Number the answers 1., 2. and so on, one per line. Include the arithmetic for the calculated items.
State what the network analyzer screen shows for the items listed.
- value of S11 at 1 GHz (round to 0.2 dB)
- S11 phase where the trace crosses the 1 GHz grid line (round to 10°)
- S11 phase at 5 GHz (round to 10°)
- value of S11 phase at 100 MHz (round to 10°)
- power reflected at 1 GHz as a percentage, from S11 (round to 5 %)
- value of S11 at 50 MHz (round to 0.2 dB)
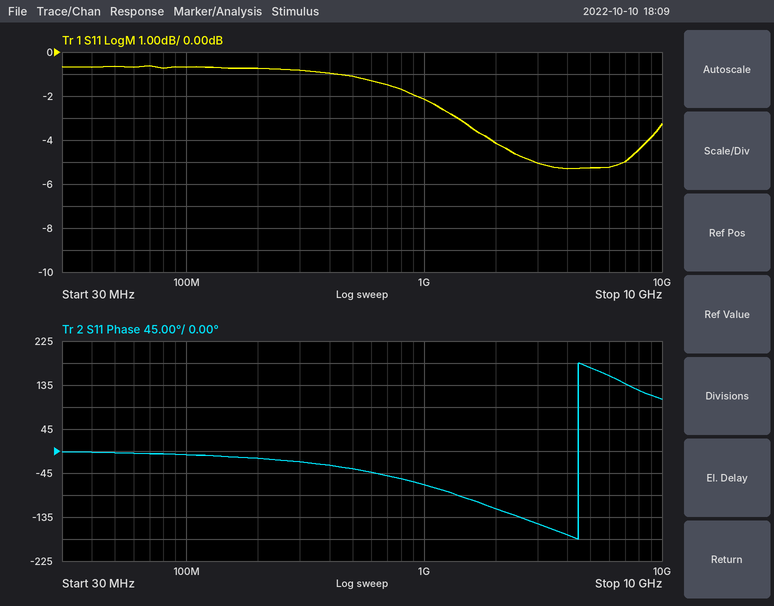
1. -2.2 dB
2. -70°
3. 170°
4. -10°
5. 10^(-2.2/10) ≈ 60 %
6. -0.6 dB
